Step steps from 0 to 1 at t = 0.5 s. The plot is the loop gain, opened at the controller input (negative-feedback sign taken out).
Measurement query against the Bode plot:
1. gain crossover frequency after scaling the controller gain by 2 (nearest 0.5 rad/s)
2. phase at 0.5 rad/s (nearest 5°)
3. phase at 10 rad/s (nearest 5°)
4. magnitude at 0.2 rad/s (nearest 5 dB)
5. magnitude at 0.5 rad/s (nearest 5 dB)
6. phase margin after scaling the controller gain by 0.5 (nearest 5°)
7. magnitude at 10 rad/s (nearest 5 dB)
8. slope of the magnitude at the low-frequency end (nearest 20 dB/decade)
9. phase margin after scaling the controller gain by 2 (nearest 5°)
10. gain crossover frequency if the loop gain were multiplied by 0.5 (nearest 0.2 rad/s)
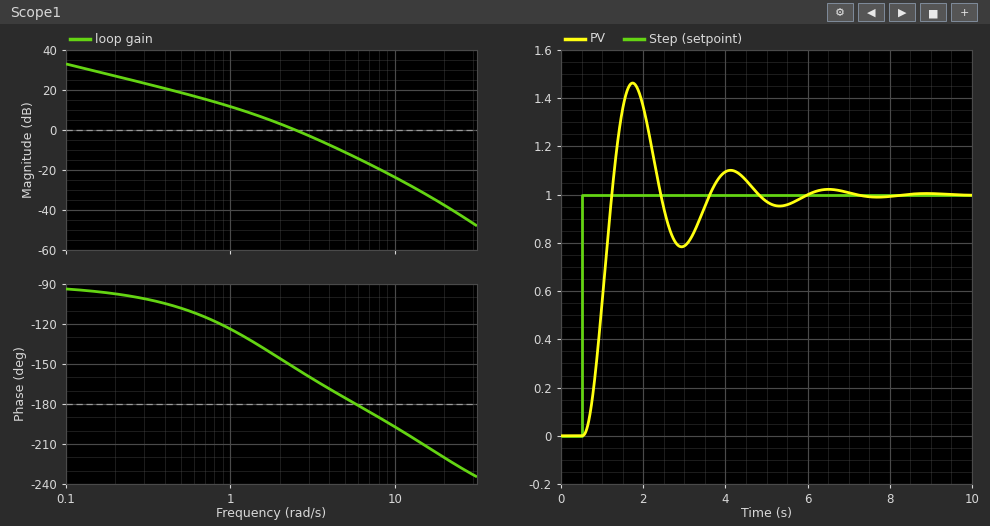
3.5 rad/s
-110°
-195°
25 dB
20 dB
40°
-25 dB
-20 dB/decade
15°
1.6 rad/s
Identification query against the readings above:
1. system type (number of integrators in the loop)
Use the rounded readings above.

1
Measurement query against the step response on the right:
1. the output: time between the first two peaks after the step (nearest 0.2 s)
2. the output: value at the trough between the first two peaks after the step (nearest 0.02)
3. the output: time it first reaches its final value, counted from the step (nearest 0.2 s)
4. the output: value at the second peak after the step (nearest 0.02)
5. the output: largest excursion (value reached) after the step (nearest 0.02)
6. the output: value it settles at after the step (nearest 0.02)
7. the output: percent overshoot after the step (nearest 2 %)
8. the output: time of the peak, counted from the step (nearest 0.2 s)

2.4 s
0.78
0.8 s
1.10
1.46
1.00
46 %
1.2 s
